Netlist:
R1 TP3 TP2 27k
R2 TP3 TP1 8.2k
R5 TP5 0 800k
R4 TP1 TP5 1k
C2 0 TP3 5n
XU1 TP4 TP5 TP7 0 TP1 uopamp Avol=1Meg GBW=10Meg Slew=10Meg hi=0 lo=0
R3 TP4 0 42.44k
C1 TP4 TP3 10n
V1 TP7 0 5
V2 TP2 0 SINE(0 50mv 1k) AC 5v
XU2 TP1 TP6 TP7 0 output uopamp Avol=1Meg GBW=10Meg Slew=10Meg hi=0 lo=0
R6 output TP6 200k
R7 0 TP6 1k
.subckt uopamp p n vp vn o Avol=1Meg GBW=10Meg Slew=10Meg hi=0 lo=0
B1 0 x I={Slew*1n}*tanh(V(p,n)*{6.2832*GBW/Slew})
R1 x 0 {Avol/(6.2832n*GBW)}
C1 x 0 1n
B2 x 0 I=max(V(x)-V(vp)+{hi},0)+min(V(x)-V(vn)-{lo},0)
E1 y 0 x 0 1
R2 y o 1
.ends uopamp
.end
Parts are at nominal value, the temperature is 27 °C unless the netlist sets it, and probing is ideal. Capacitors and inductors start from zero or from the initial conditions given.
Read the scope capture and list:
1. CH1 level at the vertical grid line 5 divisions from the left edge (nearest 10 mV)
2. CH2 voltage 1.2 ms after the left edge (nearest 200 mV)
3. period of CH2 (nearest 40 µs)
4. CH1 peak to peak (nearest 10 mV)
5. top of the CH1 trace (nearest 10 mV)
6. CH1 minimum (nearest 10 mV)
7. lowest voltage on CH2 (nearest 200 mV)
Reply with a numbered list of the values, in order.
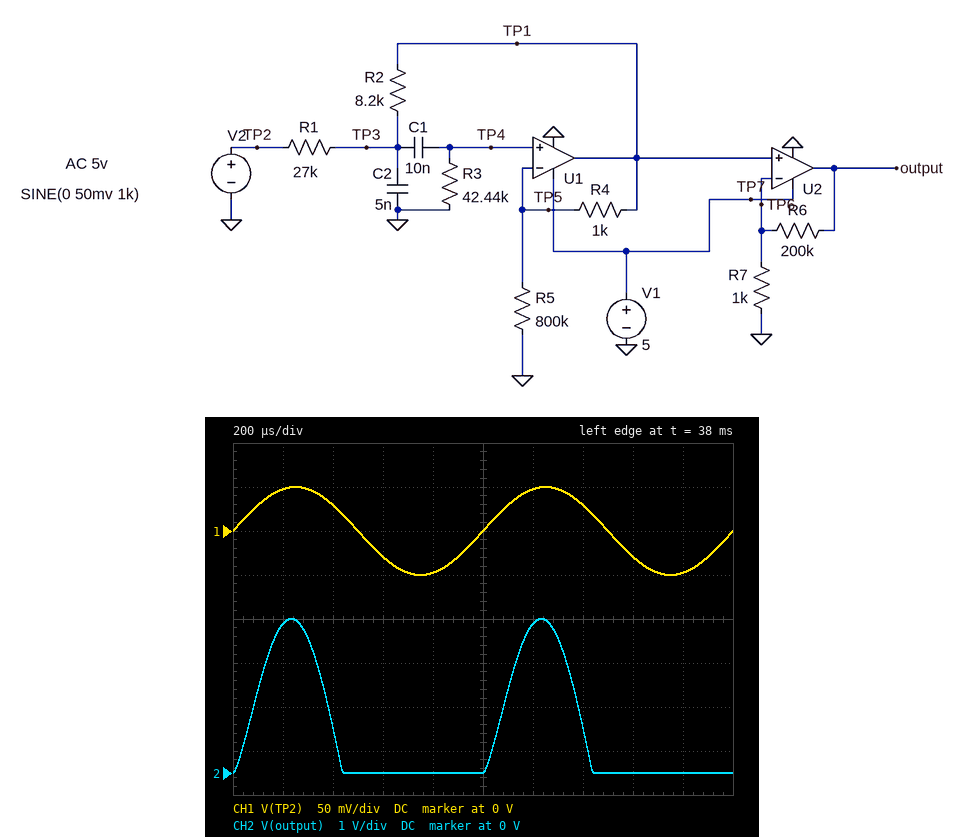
1. 0 V
2. 3.4 V
3. 1.00 ms
4. 100 mV
5. 50 mV
6. -50 mV
7. 0 V
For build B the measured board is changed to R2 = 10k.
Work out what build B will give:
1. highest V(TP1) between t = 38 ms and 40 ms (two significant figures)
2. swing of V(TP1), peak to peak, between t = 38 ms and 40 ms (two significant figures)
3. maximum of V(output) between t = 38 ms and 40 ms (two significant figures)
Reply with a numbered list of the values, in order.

1. 18 mV
2. 19 mV
3. 3.7 V
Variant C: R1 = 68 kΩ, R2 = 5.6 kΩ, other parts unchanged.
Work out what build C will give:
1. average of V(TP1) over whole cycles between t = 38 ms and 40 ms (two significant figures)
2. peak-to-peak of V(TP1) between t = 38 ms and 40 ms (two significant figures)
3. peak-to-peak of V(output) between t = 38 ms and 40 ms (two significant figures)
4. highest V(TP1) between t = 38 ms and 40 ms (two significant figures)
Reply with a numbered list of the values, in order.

1. 1.7 mV
2. 7.9 mV
3. 1.5 V
4. 7.6 mV
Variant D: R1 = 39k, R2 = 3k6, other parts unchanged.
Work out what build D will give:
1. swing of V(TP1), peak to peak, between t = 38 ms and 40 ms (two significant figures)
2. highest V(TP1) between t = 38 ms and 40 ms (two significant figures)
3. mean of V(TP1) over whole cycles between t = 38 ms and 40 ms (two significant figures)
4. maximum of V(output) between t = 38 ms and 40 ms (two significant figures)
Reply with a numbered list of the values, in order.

1. 10 mV
2. 9.8 mV
3. 2.1 mV
4. 2.0 V
